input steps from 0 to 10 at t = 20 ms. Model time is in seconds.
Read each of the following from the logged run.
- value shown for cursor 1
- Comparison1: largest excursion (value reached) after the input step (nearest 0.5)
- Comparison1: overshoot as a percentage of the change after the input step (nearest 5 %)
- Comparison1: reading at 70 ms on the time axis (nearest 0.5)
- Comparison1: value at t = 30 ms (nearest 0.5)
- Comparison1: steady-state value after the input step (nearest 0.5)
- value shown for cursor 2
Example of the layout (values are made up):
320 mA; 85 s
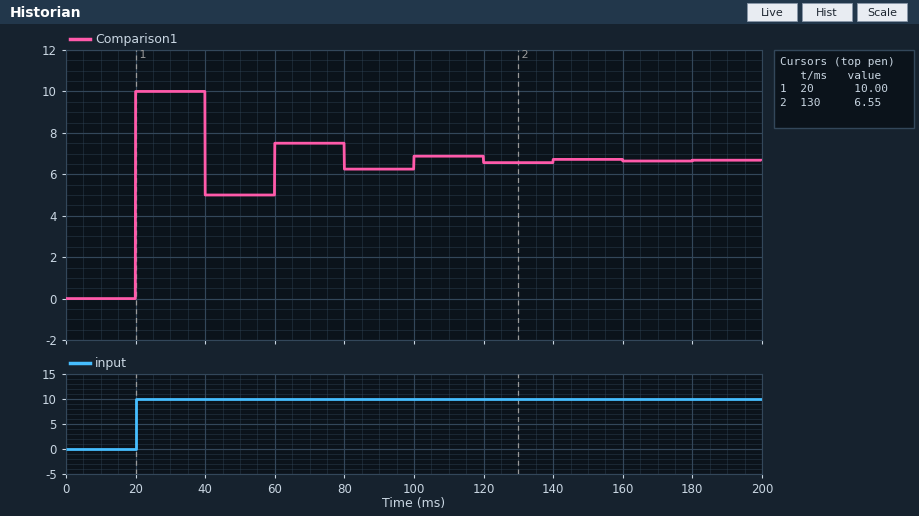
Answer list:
10.00; 10.0; 50 %; 7.5; 10.0; 6.5; 6.55
